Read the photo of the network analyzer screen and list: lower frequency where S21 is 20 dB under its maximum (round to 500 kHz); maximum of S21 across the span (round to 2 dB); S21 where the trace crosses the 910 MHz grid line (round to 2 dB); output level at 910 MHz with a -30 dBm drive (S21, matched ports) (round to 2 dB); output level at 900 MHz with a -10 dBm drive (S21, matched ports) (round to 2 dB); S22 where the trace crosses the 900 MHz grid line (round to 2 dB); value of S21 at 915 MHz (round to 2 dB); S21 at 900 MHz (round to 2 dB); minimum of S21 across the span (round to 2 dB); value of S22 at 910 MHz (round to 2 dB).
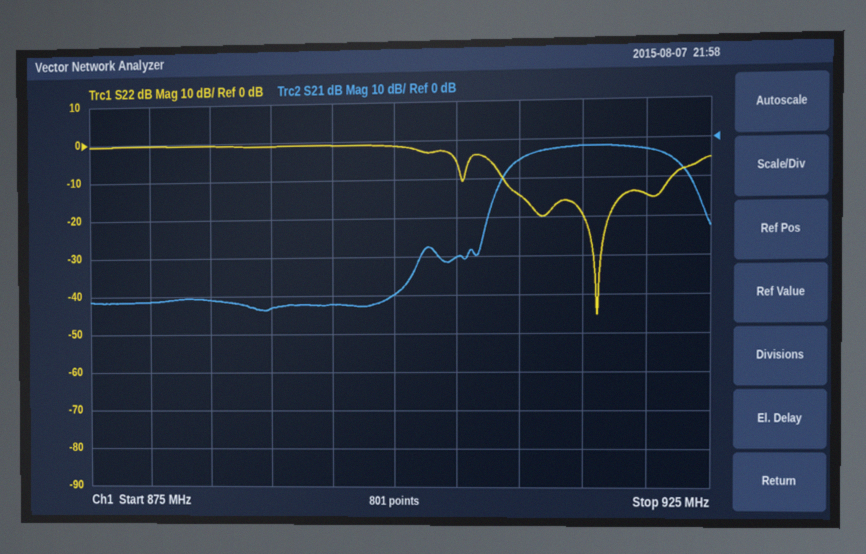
907.5 MHz
-2 dB
-6 dB
-36 dBm
-50 dBm
-2 dB
-2 dB
-40 dB
-44 dB
-14 dB
